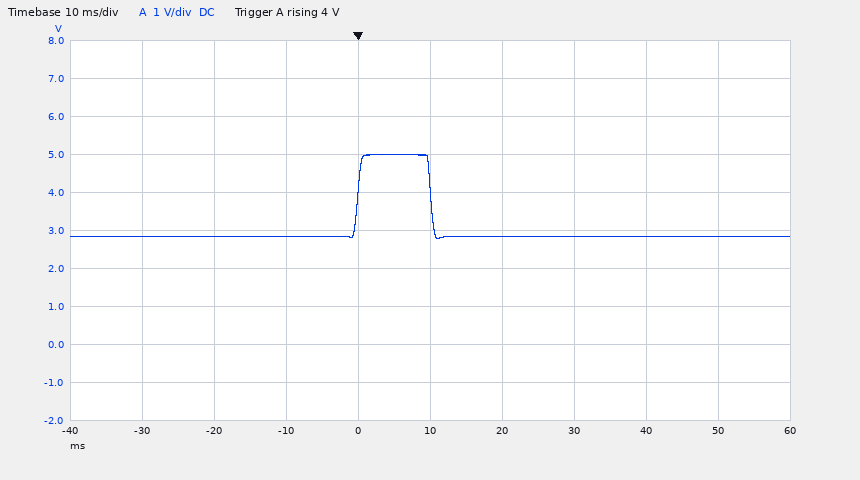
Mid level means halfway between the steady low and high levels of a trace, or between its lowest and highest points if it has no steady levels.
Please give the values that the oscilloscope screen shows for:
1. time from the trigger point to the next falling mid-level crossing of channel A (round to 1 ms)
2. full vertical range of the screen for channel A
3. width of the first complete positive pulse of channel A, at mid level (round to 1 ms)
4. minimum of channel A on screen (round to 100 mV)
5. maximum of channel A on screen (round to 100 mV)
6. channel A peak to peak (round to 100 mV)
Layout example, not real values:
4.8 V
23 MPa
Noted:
10 ms
10 V
10 ms
2.8 V
5.0 V
2.2 V
